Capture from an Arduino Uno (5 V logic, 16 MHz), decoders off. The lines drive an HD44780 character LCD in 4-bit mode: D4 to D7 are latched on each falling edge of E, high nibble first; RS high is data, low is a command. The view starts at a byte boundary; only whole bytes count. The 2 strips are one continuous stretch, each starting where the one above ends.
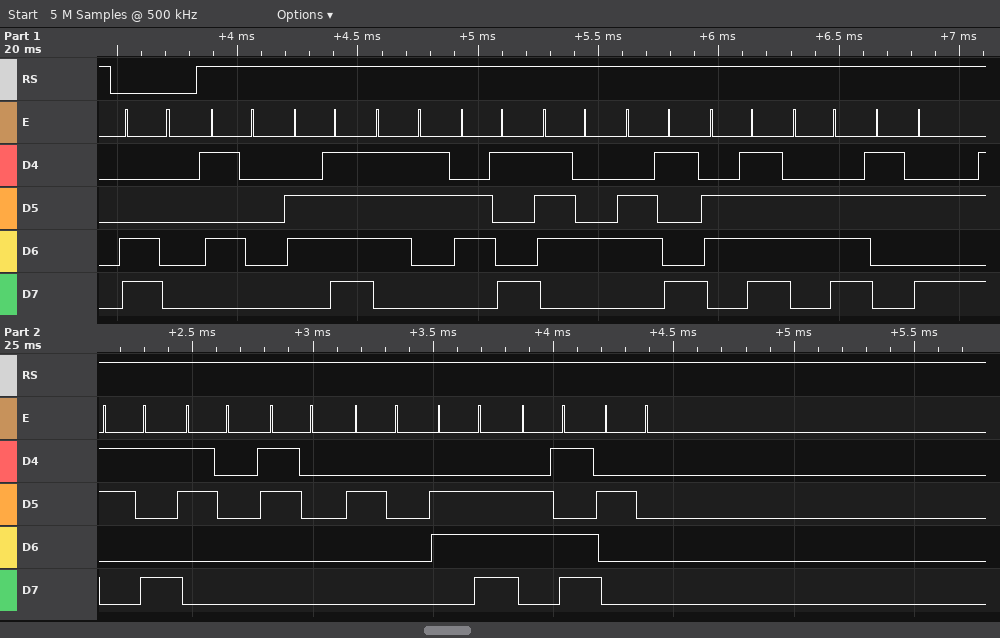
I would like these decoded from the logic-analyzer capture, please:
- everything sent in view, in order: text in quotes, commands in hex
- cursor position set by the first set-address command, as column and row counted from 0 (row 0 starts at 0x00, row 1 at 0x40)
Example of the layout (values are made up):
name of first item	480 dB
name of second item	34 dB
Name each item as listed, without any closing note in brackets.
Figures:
everything sent in view, in order: text in quotes, commands in hex	0xC0 "Position:900 nm "
cursor position set by the first set-address command, as column and row counted from 0	column 0, row 1
